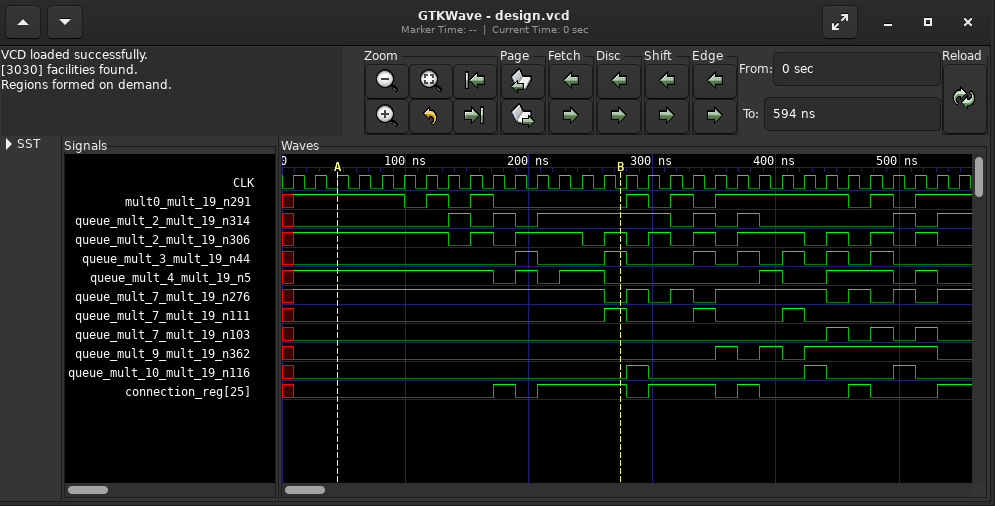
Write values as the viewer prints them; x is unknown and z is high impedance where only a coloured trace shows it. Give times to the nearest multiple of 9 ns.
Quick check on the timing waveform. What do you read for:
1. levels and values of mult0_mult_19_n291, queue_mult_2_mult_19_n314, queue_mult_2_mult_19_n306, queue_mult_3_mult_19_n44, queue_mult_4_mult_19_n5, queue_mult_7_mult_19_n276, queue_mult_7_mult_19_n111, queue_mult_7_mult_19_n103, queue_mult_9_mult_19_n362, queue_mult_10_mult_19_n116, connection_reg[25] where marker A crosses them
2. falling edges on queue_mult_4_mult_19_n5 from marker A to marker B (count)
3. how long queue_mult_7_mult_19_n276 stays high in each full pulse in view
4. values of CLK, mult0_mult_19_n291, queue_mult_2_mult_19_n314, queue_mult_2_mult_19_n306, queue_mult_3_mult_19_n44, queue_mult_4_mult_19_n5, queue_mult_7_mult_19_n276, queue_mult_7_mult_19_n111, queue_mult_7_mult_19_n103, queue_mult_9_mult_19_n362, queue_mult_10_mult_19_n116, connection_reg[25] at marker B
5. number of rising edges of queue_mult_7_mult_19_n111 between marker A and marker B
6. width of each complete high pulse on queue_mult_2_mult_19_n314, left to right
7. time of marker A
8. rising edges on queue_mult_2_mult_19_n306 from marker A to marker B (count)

mult0_mult_19_n291=1, queue_mult_2_mult_19_n314=0, queue_mult_2_mult_19_n306=1, queue_mult_3_mult_19_n44=0, queue_mult_4_mult_19_n5=1, queue_mult_7_mult_19_n276=1, queue_mult_7_mult_19_n111=0, queue_mult_7_mult_19_n103=0, queue_mult_9_mult_19_n362=0, queue_mult_10_mult_19_n116=0, connection_reg[25]=0
3
18 ns, 18 ns, 90 ns, 18 ns, 18 ns
CLK=0, mult0_mult_19_n291=0, queue_mult_2_mult_19_n314=1, queue_mult_2_mult_19_n306=1, queue_mult_3_mult_19_n44=1, queue_mult_4_mult_19_n5=0, queue_mult_7_mult_19_n276=0, queue_mult_7_mult_19_n111=1, queue_mult_7_mult_19_n103=0, queue_mult_9_mult_19_n362=0, queue_mult_10_mult_19_n116=0, connection_reg[25]=1
1
18 ns, 18 ns, 108 ns, 18 ns, 18 ns, 18 ns
45 ns
3
